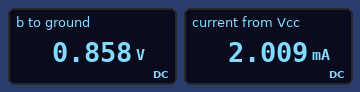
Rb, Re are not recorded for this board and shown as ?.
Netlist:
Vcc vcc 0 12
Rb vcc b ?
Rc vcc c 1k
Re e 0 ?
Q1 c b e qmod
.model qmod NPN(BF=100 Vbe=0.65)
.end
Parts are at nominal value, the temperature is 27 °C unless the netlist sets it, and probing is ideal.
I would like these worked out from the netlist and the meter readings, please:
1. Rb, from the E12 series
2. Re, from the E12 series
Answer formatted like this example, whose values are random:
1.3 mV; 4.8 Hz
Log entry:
560 kΩ; 33 Ω
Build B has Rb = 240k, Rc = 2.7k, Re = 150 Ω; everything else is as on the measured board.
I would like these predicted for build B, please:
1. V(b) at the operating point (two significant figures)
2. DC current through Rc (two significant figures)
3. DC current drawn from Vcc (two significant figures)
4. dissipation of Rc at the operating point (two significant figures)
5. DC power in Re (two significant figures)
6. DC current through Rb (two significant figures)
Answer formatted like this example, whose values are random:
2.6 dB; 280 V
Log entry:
1.4 V; 4.1 mA; 4.2 mA; 46 mW; 2.6 mW; 44 µA
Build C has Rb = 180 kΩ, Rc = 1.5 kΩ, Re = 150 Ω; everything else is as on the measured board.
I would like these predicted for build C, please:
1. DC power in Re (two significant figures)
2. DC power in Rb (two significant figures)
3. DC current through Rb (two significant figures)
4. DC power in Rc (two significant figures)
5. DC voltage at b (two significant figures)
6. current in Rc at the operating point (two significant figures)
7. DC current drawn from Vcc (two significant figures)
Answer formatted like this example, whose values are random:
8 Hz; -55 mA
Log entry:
5.0 mW; 590 µW; 57 µA; 49 mW; 1.7 V; 5.7 mA; 5.8 mA
